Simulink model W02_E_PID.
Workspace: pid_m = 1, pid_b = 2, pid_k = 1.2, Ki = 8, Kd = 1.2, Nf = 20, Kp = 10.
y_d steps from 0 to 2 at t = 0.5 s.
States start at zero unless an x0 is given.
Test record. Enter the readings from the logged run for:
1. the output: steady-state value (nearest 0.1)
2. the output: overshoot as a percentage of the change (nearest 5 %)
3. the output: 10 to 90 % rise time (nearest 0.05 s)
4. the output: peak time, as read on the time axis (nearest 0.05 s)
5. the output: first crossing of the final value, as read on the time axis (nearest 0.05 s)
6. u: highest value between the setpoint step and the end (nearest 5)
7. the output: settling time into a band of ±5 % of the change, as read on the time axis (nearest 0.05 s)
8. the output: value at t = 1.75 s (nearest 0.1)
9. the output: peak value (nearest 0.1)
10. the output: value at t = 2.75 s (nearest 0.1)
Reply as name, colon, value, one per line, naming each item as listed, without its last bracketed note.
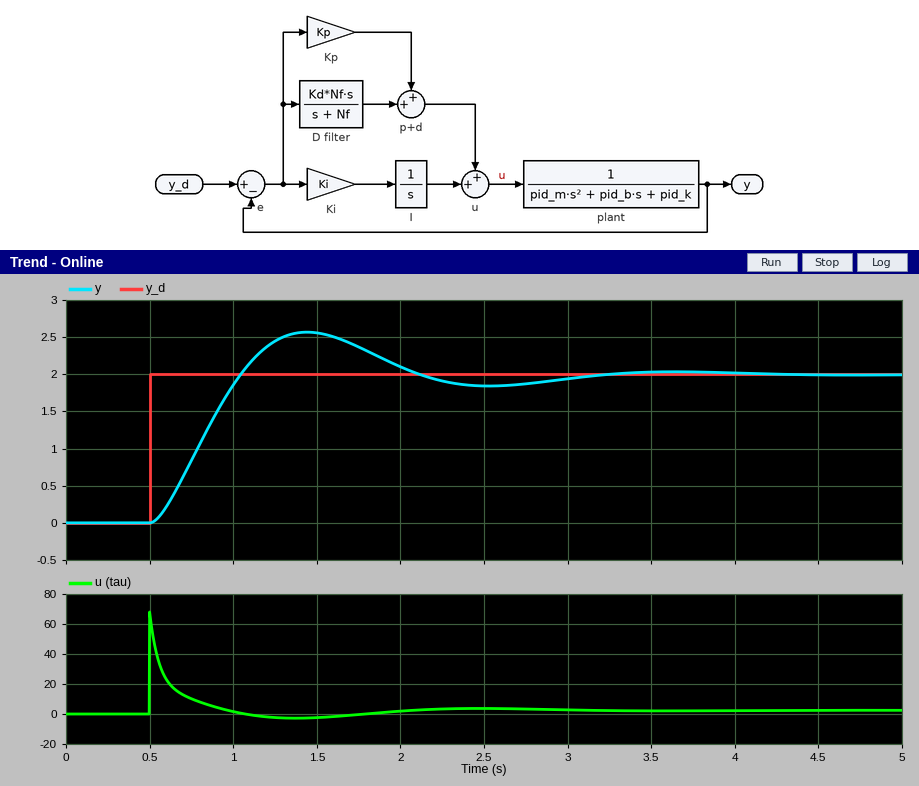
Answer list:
the output: steady-state value: 2.0
the output: overshoot as a percentage of the change: 30 %
the output: 10 to 90 % rise time: 0.40 s
the output: peak time, as read on the time axis: 1.45 s
the output: first crossing of the final value, as read on the time axis: 1.05 s
u: highest value between the setpoint step and the end: 70
the output: settling time into a band of ±5 % of the change, as read on the time axis: 2.85 s
the output: value at t = 1.75 s: 2.4
the output: peak value: 2.6
the output: value at t = 2.75 s: 1.9
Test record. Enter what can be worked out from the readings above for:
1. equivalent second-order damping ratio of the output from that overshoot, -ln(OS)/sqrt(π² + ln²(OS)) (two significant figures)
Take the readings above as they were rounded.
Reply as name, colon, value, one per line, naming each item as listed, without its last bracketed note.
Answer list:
equivalent second-order damping ratio of the output from that overshoot, -ln(OS)/sqrt(π² + ln²(OS)): 0.36
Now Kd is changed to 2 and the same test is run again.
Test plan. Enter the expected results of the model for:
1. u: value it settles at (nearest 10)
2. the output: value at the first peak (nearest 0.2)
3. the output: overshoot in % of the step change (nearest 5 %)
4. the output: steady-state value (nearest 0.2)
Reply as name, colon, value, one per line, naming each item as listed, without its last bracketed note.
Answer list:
u: value it settles at: 0
the output: value at the first peak: 2.4
the output: overshoot in % of the step change: 20 %
the output: steady-state value: 2.0
